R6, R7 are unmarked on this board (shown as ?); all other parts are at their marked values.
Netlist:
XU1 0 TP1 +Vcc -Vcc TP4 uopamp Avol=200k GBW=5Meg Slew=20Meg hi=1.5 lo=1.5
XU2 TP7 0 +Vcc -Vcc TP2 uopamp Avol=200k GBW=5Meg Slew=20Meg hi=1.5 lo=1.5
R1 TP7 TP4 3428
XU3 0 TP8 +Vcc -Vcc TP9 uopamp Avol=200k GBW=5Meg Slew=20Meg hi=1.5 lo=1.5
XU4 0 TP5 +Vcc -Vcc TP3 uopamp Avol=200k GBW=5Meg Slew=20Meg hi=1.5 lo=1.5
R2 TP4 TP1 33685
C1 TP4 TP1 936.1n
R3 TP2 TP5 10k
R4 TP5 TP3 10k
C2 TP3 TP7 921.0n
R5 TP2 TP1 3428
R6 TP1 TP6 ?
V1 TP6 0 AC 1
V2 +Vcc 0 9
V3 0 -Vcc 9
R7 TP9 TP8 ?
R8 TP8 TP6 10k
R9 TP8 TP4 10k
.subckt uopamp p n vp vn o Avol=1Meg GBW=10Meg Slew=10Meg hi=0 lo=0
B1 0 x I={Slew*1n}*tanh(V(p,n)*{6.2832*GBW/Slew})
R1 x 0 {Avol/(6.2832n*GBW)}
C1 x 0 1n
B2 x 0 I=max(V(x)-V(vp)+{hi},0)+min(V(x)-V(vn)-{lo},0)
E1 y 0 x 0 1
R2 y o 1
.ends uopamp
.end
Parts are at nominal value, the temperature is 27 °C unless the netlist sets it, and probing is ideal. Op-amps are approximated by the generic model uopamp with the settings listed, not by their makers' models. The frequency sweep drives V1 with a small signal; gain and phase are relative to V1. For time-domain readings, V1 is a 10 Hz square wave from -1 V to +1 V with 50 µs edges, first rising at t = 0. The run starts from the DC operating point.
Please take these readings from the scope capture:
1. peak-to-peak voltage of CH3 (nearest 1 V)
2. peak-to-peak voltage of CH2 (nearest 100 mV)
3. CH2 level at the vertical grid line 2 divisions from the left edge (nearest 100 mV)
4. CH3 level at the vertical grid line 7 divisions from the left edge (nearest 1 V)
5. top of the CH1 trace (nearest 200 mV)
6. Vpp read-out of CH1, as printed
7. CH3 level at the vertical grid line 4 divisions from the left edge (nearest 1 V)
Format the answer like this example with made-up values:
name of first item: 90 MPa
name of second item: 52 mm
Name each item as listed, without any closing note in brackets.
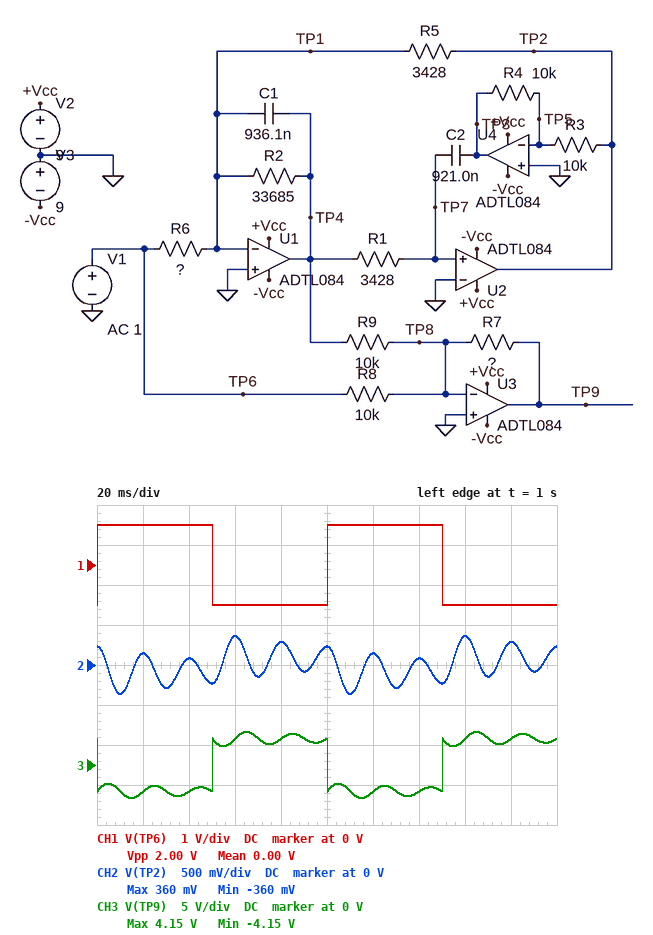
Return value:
peak-to-peak voltage of CH3: 8 V
peak-to-peak voltage of CH2: 700 mV
CH2 level at the vertical grid line 2 divisions from the left edge: 100 mV
CH3 level at the vertical grid line 7 divisions from the left edge: -3 V
top of the CH1 trace: 1.0 V
Vpp read-out of CH1, as printed: 2.00 V
CH3 level at the vertical grid line 4 divisions from the left edge: 3 V
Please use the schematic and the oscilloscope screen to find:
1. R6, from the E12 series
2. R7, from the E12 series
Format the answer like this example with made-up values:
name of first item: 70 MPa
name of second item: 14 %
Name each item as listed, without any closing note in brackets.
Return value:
R6, from the E12 series: 39 kΩ
R7, from the E12 series: 33 kΩ
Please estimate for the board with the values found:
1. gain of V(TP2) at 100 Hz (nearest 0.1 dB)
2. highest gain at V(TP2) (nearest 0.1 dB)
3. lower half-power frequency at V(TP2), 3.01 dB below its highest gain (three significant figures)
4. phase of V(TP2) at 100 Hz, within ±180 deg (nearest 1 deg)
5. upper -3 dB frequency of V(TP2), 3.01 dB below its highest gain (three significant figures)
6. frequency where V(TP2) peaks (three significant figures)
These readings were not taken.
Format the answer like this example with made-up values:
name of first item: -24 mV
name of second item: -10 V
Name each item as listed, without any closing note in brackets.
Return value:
gain of V(TP2) at 100 Hz: -30.7 dB
highest gain at V(TP2): -1.2 dB
lower half-power frequency at V(TP2), 3.01 dB below its highest gain: 47.3 Hz
phase of V(TP2) at 100 Hz, within ±180 deg: 4 deg
upper -3 dB frequency of V(TP2), 3.01 dB below its highest gain: 52.3 Hz
frequency where V(TP2) peaks: 49.9 Hz
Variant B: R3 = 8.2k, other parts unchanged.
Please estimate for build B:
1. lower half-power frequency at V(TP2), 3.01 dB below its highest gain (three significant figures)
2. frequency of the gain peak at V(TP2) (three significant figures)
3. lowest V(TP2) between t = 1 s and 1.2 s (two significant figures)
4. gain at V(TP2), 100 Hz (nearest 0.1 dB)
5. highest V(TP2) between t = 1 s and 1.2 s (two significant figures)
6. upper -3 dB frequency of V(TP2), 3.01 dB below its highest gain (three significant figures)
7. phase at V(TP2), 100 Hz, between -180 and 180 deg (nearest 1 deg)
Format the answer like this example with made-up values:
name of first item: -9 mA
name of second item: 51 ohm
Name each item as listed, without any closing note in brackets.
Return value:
lower half-power frequency at V(TP2), 3.01 dB below its highest gain: 42.5 Hz
frequency of the gain peak at V(TP2): 45.1 Hz
lowest V(TP2) between t = 1 s and 1.2 s: -220 mV
gain at V(TP2), 100 Hz: -32.9 dB
highest V(TP2) between t = 1 s and 1.2 s: 220 mV
upper -3 dB frequency of V(TP2), 3.01 dB below its highest gain: 47.6 Hz
phase at V(TP2), 100 Hz, between -180 and 180 deg: 4 deg
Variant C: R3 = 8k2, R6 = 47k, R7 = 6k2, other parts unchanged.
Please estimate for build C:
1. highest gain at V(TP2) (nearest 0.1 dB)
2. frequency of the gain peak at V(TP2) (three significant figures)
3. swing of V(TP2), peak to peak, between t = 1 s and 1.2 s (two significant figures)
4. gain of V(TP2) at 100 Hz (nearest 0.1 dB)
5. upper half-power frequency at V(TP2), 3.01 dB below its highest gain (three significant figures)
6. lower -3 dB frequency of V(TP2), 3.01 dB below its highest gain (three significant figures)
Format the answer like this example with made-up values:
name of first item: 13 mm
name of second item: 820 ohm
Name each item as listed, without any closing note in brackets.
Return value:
highest gain at V(TP2): -3.7 dB
frequency of the gain peak at V(TP2): 45.1 Hz
swing of V(TP2), peak to peak, between t = 1 s and 1.2 s: 370 mV
gain of V(TP2) at 100 Hz: -34.5 dB
upper half-power frequency at V(TP2), 3.01 dB below its highest gain: 47.6 Hz
lower -3 dB frequency of V(TP2), 3.01 dB below its highest gain: 42.5 Hz
